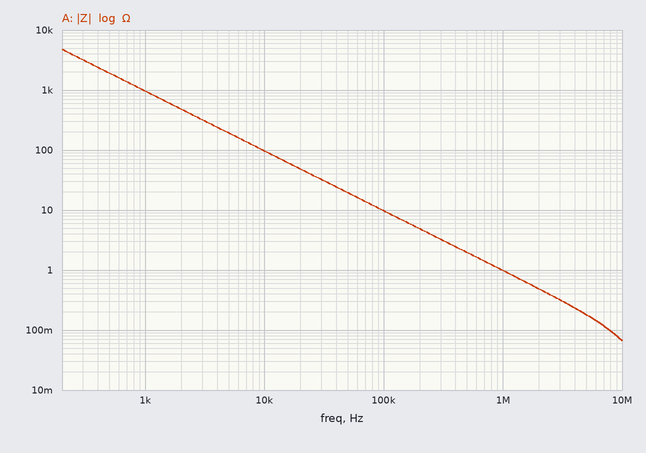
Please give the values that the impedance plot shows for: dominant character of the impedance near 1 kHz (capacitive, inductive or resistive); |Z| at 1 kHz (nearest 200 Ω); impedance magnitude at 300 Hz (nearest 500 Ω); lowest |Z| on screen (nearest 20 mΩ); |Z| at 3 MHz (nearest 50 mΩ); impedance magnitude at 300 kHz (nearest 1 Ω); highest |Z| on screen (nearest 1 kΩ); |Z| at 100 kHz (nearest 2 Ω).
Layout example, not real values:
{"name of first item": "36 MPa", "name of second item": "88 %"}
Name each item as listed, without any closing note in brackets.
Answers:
{"dominant character of the impedance near 1 kHz": "capacitive", "|Z| at 1 kHz": "1.0 kΩ", "impedance magnitude at 300 Hz": "3.0 kΩ", "lowest |Z| on screen": "60 mΩ", "|Z| at 3 MHz": "300 mΩ", "impedance magnitude at 300 kHz": "3 Ω", "highest |Z| on screen": "5 kΩ", "|Z| at 100 kHz": "10 Ω"}
